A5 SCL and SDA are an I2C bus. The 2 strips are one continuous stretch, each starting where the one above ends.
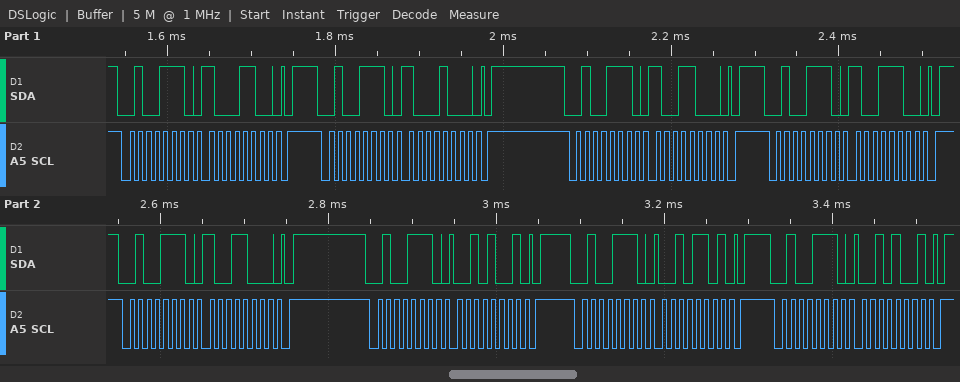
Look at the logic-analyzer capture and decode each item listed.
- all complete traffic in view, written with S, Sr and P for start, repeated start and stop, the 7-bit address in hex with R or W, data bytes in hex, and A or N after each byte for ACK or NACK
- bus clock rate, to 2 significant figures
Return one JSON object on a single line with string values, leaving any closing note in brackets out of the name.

{"all complete traffic in view, written with S, Sr and P for start, repeated start and stop, the 7-bit address in hex with R or W, data bytes in hex, and A or N after each byte for ACK or NACK": "S 27W A 8C A P S 27W A 88 A P S 27W A 98 A P S 27W A 9C A P S 27W A 98 A P S 27W A 29 A P S 27W A 2D A P S 27W A 29 A P", "bus clock rate, to 2 significant figures": "100 kHz"}
